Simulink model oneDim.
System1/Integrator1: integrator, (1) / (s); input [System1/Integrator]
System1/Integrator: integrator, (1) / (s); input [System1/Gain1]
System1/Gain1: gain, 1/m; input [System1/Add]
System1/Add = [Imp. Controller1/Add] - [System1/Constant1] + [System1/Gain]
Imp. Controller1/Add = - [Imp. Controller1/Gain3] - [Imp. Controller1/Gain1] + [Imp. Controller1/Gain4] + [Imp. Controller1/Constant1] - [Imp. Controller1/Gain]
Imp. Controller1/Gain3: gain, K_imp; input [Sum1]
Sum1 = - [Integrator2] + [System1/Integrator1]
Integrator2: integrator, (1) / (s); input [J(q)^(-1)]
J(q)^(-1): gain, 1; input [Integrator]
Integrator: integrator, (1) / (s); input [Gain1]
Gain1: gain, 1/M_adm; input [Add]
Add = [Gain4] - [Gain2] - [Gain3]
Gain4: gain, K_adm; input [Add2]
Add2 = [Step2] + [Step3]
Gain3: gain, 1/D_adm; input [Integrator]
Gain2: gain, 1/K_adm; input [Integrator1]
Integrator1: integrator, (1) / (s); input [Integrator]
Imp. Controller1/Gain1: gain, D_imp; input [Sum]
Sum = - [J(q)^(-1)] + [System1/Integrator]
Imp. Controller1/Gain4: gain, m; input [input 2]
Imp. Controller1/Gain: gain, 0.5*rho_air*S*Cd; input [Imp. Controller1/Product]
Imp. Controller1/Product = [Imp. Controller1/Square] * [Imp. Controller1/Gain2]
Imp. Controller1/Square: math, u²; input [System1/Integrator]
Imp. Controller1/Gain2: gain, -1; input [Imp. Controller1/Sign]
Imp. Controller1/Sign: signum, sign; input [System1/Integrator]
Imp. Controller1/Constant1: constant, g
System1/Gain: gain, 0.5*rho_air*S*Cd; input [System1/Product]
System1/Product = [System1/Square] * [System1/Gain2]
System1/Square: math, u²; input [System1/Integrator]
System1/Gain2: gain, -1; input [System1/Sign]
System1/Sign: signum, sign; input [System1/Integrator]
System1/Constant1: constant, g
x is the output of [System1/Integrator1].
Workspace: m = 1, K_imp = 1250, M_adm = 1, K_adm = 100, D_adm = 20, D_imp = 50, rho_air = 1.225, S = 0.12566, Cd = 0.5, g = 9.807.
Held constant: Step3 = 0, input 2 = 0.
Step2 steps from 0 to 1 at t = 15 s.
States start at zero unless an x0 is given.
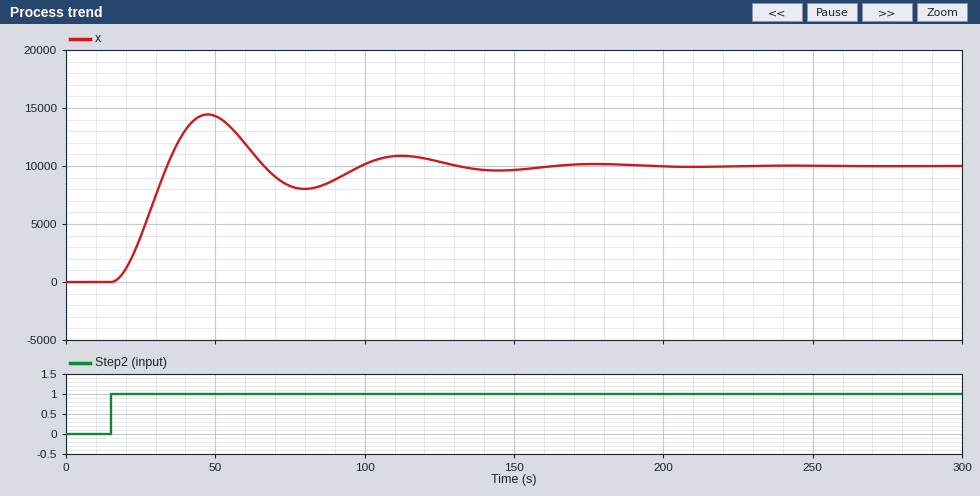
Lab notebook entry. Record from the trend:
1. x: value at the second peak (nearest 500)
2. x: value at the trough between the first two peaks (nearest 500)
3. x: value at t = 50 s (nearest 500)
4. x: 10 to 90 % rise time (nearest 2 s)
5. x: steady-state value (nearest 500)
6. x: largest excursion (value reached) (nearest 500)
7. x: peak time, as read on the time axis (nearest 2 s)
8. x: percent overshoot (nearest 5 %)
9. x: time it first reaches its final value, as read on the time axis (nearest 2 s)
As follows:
11000
8000
14500
12 s
10000
14500
48 s
45 %
34 s
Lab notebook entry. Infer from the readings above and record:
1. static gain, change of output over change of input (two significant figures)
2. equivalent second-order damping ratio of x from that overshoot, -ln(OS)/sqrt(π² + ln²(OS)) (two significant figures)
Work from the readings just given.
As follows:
10000
0.25
